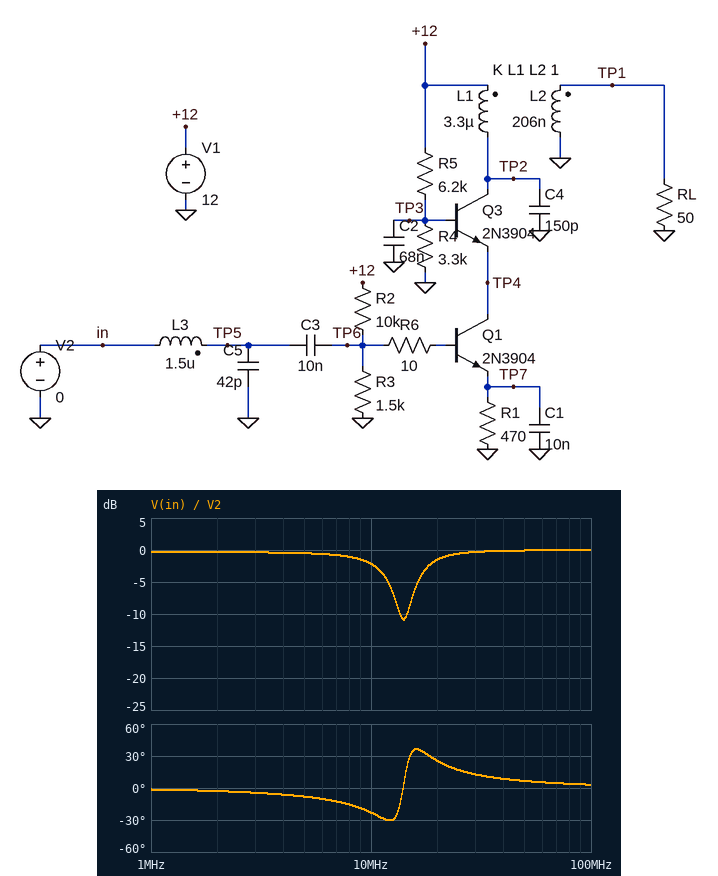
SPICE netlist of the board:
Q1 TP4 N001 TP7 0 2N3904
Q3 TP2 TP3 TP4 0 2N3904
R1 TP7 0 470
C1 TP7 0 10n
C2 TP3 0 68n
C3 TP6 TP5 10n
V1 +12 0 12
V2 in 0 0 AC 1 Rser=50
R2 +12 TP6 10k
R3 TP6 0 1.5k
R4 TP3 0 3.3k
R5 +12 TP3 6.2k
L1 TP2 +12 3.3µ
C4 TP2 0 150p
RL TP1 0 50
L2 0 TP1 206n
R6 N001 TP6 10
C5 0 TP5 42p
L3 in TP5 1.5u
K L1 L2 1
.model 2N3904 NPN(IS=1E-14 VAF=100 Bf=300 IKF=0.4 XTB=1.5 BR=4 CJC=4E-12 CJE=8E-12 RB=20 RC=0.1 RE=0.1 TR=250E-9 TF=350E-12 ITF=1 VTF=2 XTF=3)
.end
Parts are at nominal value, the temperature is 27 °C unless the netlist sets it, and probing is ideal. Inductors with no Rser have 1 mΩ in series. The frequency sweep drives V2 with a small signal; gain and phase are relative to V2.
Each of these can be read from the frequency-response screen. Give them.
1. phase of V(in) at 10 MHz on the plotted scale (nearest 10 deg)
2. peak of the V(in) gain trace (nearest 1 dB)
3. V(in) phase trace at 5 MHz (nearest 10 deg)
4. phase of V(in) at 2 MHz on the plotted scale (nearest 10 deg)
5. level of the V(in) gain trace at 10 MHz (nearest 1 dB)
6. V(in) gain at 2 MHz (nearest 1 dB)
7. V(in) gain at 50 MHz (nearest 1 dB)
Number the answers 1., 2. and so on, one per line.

1. -20 deg
2. 0 dB
3. -10 deg
4. 0 deg
5. -2 dB
6. 0 dB
7. 0 dB
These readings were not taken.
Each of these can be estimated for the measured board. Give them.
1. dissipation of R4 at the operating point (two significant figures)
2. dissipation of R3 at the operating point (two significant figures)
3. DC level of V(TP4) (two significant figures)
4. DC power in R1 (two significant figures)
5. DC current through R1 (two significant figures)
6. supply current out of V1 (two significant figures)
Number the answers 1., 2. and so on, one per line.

1. 5.2 mW
2. 1.6 mW
3. 3.5 V
4. 1.7 mW
5. 1.9 mA
6. 4.2 mA
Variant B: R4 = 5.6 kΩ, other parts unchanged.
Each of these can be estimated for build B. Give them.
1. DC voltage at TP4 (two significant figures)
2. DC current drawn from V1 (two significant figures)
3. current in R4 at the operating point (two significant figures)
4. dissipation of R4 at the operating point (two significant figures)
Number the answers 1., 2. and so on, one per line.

1. 5.0 V
2. 3.9 mA
3. 1.0 mA
4. 5.8 mW
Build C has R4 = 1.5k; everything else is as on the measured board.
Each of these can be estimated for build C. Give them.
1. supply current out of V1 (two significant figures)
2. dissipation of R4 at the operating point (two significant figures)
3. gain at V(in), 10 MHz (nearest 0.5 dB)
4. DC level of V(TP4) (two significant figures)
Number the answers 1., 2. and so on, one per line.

1. 4.5 mA
2. 3.6 mW
3. -2.5 dB
4. 1.7 V
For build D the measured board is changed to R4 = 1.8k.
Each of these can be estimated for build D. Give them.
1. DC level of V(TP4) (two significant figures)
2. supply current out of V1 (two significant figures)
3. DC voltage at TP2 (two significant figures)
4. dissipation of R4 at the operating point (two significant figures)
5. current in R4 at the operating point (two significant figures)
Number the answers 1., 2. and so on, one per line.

1. 2.0 V
2. 4.4 mA
3. 12 V
4. 4.0 mW
5. 1.5 mA
